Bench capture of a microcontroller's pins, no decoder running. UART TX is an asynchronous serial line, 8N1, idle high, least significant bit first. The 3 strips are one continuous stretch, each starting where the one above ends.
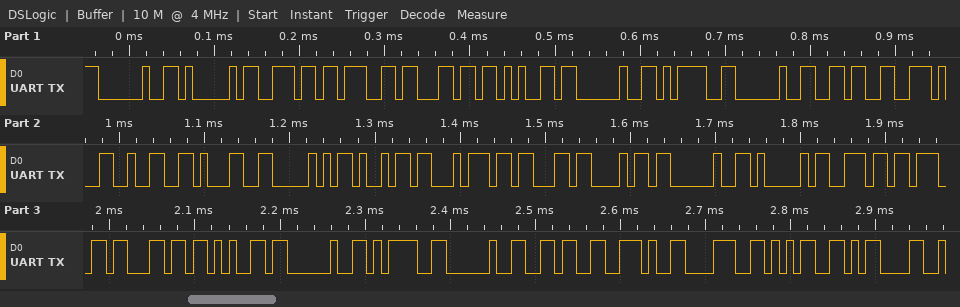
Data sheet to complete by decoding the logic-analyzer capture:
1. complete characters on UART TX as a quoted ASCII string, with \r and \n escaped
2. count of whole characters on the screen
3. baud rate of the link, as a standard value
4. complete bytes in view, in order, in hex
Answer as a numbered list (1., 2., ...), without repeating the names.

1. " Angle = 6.21Pitch Angle = 6.85\r"
2. 32
3. 115200 baud
4. 0x20 0x41 0x6E 0x67 0x6C 0x65 0x20 0x3D 0x20 0x36 0x2E 0x32 0x31 0x50 0x69 0x74 0x63 0x68 0x20 0x41 0x6E 0x67 0x6C 0x65 0x20 0x3D 0x20 0x36 0x2E 0x38 0x35 0x0D
